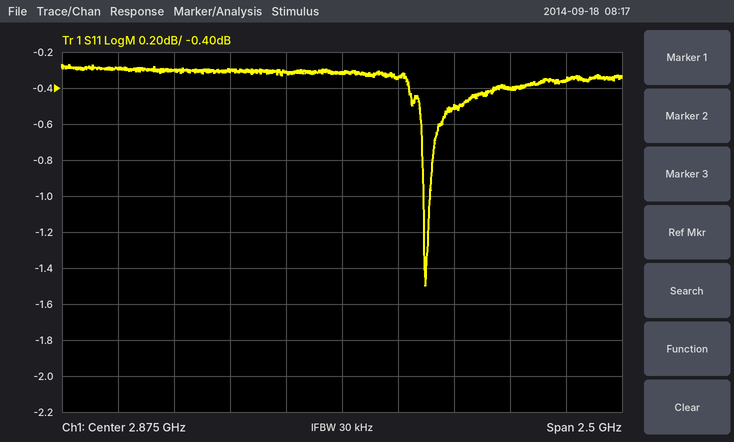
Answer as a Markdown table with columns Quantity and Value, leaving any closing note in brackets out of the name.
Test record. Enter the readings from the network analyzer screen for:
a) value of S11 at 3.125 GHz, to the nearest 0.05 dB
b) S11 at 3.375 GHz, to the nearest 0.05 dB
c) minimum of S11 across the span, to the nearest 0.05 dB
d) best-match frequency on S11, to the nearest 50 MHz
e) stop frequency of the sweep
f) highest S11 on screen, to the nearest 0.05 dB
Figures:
| Quantity | Value |
|---|---|
| value of S11 at 3.125 GHz, to the nearest 0.05 dB | -0.35 dB |
| S11 at 3.375 GHz, to the nearest 0.05 dB | -0.50 dB |
| minimum of S11 across the span, to the nearest 0.05 dB | -1.50 dB |
| best-match frequency on S11, to the nearest 50 MHz | 3.25 GHz |
| stop frequency of the sweep | 4.125 GHz |
| highest S11 on screen, to the nearest 0.05 dB | -0.25 dB |
